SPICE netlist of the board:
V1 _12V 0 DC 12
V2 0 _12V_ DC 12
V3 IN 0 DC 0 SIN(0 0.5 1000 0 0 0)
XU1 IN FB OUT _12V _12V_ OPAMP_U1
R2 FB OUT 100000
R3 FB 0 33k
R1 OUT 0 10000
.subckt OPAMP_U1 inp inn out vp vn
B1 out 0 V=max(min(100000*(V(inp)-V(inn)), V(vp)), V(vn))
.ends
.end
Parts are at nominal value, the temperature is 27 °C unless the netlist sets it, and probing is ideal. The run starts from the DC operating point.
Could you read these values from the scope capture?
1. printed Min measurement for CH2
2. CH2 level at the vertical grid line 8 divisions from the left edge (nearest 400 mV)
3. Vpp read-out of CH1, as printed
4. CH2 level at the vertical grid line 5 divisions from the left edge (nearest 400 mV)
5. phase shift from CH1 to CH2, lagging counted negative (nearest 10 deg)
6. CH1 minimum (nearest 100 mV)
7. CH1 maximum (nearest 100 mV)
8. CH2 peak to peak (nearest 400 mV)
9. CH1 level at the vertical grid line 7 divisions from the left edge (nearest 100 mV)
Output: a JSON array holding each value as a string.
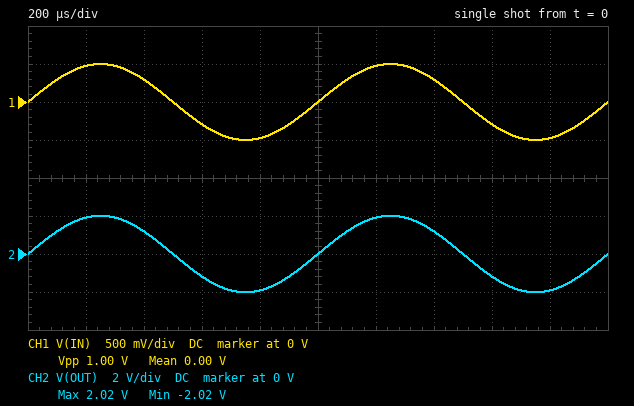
["-2.02 V", "-1.2 V", "1.00 V", "0 V", "0 deg", "-500 mV", "500 mV", "4.0 V", "300 mV"]
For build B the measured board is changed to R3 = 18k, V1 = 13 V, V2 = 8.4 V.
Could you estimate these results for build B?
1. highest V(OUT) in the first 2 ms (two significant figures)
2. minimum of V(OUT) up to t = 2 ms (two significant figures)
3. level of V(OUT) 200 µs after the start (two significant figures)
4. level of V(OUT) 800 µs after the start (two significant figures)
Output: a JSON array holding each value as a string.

["3.3 V", "-3.3 V", "3.1 V", "-3.1 V"]
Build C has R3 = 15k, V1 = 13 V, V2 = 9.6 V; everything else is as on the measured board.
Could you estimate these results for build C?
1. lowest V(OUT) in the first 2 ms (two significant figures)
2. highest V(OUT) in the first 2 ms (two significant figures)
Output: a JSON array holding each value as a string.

["-3.8 V", "3.8 V"]
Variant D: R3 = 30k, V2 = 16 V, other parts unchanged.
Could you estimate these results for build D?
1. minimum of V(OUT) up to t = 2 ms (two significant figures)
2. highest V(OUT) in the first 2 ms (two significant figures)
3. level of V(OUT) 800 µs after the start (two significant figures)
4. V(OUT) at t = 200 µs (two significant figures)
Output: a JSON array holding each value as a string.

["-2.2 V", "2.2 V", "-2.1 V", "2.1 V"]
